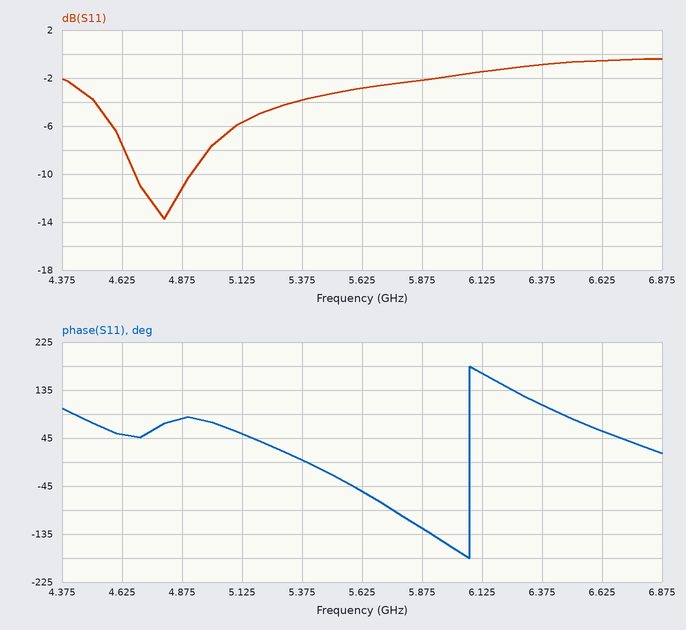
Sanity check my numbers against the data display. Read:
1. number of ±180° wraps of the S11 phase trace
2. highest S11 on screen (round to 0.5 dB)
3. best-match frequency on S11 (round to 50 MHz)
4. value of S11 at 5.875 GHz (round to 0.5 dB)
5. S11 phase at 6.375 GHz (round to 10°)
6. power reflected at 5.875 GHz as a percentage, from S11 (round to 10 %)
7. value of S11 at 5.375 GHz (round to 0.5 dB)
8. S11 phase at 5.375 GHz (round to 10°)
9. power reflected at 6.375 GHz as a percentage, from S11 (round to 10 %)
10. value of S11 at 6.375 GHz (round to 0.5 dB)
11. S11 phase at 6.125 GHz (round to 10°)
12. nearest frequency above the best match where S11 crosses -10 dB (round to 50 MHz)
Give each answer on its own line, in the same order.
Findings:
1
-0.5 dB
4.80 GHz
-2.0 dB
110°
60 %
-4.0 dB
0°
80 %
-1.0 dB
170°
4.90 GHz
